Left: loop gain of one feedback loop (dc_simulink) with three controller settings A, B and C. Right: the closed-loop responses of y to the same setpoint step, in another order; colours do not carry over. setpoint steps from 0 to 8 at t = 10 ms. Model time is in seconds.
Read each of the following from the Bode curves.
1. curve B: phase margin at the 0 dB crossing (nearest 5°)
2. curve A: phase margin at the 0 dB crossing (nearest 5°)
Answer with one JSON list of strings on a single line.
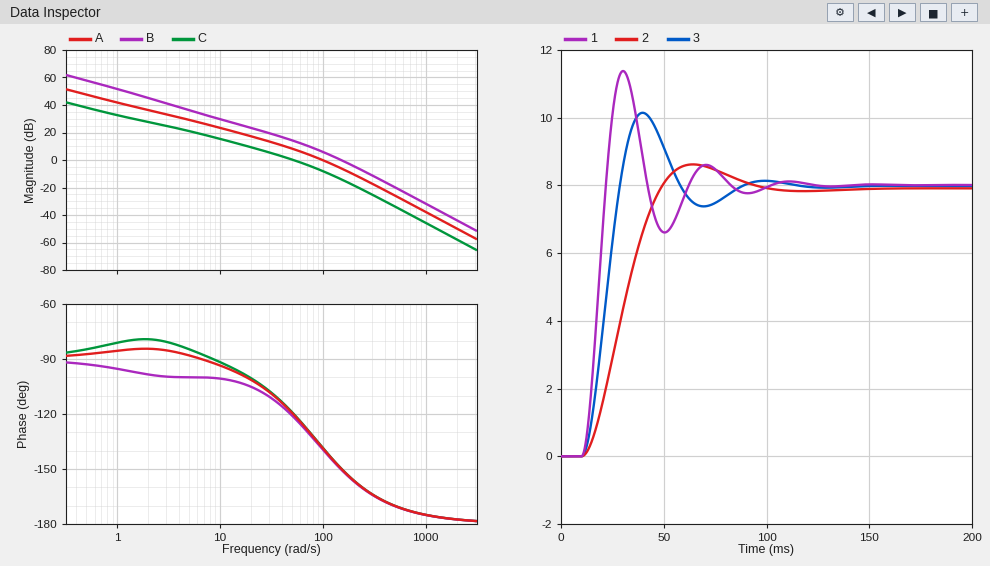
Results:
["30°", "40°"]
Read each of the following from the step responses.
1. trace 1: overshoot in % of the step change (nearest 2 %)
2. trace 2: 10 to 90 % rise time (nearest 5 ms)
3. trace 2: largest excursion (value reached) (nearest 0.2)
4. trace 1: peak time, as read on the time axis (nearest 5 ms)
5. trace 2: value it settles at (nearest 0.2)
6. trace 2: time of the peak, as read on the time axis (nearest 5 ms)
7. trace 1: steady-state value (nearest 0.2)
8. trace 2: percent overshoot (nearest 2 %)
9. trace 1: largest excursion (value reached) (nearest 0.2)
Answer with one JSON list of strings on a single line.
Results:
["42 %", "25 ms", "8.6", "30 ms", "8.0", "65 ms", "8.0", "8 %", "11.4"]
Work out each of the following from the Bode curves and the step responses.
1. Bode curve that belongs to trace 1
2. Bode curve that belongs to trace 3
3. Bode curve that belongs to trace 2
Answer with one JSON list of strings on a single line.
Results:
["B", "A", "C"]
